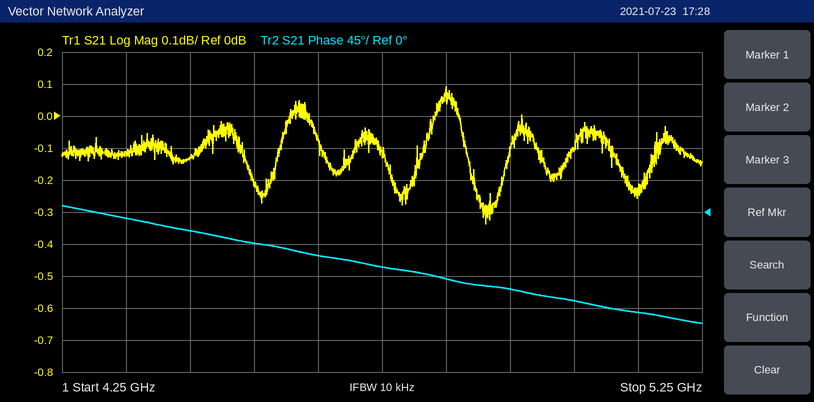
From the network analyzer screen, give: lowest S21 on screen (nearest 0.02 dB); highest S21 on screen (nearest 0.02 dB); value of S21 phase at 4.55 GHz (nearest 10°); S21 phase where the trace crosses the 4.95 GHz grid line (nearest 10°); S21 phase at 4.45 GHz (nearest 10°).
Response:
-0.34 dB
0.10 dB
-40°
-110°
-30°
